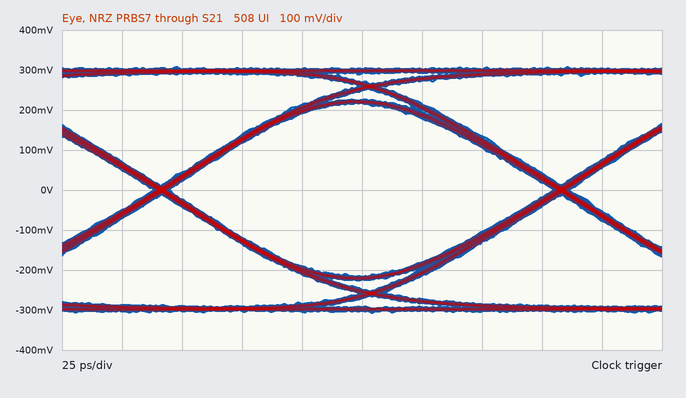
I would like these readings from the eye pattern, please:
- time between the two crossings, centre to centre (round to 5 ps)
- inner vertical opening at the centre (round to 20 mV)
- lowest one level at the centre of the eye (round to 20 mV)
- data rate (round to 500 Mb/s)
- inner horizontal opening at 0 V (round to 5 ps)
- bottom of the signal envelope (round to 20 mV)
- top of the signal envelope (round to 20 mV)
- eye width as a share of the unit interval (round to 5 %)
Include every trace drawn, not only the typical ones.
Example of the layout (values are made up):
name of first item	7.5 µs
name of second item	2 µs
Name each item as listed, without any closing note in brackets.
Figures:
time between the two crossings, centre to centre	165 ps
inner vertical opening at the centre	440 mV
lowest one level at the centre of the eye	220 mV
data rate	6.0 Gb/s
inner horizontal opening at 0 V	160 ps
bottom of the signal envelope	-300 mV
top of the signal envelope	300 mV
eye width as a share of the unit interval	95 %
